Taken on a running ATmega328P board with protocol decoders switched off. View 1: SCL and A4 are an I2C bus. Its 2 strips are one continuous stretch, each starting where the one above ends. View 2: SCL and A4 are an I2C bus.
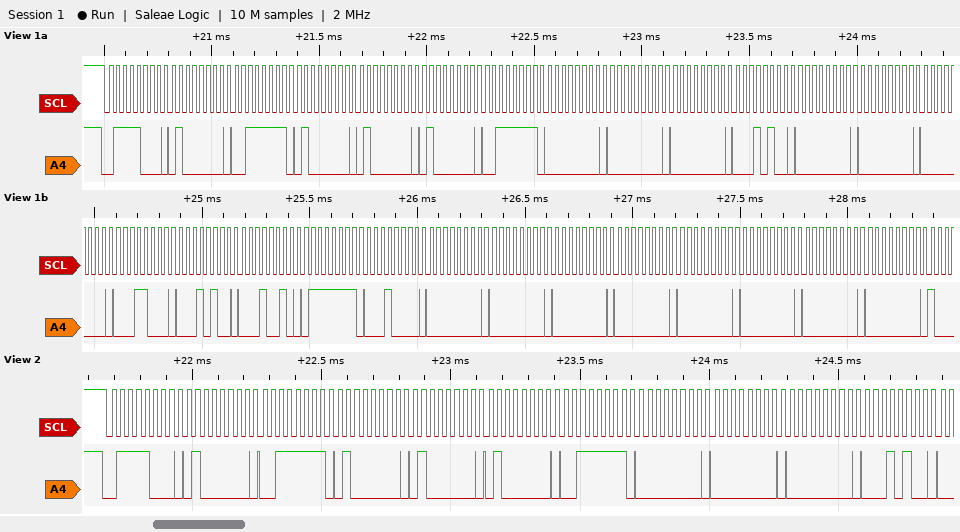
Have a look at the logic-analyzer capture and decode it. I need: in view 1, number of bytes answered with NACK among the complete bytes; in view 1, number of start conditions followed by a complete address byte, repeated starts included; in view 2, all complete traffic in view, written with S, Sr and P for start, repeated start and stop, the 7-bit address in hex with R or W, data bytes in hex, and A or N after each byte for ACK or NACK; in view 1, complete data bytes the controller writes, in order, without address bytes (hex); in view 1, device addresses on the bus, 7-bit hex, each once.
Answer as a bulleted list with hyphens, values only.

- 0
- 1
- S 3CW A 40 A 3F A 40 A 40 A 40 A 3F A 00 A 00 A 00 A 14 A
- 40 3F 40 40 40 3F 00 00 00 14 00 00 00 18 14 12 7F 10 00 00 00 00 00 00 00 00
- 0x3C
